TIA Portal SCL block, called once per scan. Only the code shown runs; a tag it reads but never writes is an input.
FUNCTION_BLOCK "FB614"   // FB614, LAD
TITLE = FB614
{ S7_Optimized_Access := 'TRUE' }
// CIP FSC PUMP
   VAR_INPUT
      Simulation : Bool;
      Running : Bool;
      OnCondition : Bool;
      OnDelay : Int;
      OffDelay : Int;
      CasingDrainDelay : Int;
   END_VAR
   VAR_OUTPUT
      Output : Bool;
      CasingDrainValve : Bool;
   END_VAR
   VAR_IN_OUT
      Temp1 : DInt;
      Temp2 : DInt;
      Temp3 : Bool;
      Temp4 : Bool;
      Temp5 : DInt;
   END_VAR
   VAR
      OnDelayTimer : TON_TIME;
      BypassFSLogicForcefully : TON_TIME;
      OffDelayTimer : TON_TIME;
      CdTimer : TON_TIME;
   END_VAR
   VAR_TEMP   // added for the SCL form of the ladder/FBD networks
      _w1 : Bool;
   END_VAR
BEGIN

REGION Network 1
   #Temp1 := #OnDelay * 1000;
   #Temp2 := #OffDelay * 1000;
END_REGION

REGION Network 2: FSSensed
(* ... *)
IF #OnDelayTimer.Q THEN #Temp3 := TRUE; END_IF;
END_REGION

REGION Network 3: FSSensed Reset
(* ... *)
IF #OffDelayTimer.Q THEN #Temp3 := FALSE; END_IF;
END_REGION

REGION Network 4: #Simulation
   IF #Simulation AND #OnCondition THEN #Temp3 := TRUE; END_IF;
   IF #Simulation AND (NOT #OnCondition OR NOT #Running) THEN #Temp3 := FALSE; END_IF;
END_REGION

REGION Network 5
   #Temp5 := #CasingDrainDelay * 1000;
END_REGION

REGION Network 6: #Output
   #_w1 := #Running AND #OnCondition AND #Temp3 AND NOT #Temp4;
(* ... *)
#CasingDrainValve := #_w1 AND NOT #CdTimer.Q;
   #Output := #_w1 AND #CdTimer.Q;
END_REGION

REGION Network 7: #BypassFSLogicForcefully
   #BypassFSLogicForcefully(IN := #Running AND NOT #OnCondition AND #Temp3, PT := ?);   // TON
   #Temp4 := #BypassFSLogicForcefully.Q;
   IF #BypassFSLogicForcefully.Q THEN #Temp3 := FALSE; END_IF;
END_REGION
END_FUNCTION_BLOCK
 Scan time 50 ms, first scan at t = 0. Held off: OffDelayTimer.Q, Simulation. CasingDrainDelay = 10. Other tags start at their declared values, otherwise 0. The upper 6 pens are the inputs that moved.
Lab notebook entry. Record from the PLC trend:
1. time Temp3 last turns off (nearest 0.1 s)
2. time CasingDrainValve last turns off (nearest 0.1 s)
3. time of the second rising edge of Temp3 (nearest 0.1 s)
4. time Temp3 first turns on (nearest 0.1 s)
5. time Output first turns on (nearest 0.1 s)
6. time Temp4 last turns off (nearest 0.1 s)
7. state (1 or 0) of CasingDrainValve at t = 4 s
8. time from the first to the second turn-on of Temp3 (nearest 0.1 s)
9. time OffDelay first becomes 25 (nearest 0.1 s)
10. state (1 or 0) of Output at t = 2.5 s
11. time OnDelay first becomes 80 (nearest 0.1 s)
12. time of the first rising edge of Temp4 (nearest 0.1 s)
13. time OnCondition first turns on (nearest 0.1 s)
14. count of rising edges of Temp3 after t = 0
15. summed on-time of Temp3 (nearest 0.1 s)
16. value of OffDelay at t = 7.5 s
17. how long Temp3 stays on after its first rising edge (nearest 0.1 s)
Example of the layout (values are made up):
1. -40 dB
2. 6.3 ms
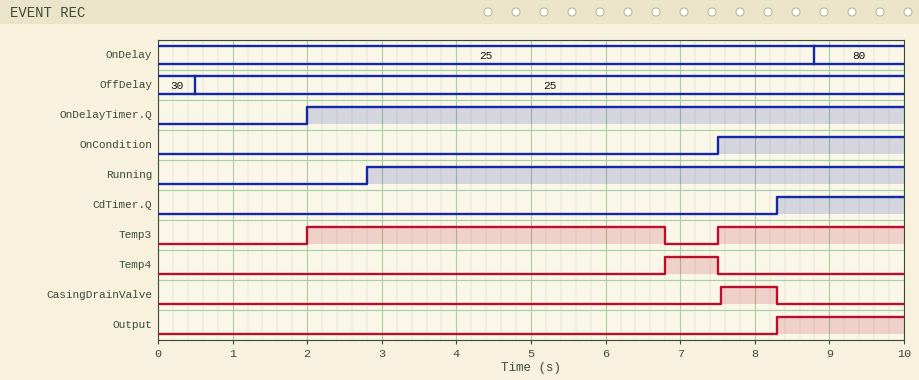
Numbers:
1. 6.8 s
2. 8.3 s
3. 7.5 s
4. 2.0 s
5. 8.3 s
6. 7.5 s
7. 0
8. 5.5 s
9. 0.5 s
10. 0
11. 8.8 s
12. 6.8 s
13. 7.5 s
14. 2
15. 7.3 s
16. 25
17. 4.8 s
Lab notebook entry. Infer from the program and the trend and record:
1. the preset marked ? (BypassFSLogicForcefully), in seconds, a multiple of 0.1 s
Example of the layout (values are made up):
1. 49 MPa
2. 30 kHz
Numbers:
1. 4.0 s
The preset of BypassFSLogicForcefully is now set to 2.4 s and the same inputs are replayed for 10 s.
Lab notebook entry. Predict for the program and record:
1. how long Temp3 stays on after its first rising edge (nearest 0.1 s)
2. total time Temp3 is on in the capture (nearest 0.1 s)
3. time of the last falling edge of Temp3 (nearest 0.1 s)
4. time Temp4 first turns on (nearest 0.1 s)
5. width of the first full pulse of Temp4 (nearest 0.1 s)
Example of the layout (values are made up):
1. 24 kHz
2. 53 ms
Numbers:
1. 3.2 s
2. 5.7 s
3. 5.2 s
4. 5.2 s
5. 2.3 s
